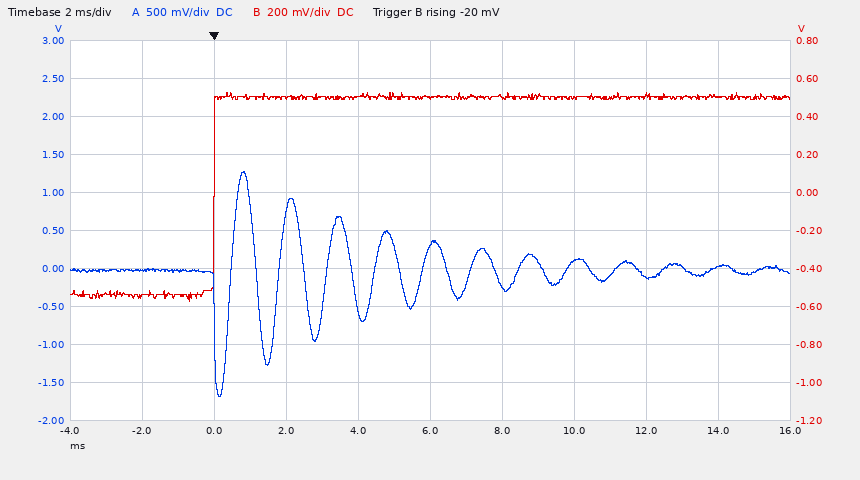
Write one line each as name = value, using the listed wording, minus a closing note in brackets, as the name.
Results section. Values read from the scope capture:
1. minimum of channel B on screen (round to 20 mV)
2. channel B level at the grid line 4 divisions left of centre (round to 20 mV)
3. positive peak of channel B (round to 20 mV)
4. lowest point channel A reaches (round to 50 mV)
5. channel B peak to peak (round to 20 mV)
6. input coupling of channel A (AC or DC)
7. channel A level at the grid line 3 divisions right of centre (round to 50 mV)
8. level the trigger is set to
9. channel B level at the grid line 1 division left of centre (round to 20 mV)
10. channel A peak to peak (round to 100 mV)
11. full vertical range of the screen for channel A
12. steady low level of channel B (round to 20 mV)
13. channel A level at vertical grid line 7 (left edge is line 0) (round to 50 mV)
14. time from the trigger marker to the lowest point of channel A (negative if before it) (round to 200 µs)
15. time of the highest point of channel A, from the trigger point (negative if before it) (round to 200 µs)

minimum of channel B on screen = -580 mV
channel B level at the grid line 4 divisions left of centre = -540 mV
positive peak of channel B = 520 mV
lowest point channel A reaches = -1.70 V
channel B peak to peak = 1.10 V
input coupling of channel A = DC
channel A level at the grid line 3 divisions right of centre = -100 mV
level the trigger is set to = -20 mV
channel B level at the grid line 1 division left of centre = 500 mV
channel A peak to peak = 3.00 V
full vertical range of the screen for channel A = 5 V
steady low level of channel B = -540 mV
channel A level at vertical grid line 7 (left edge is line 0) = 100 mV
time from the trigger marker to the lowest point of channel A (negative if before it) = +200 µs
time of the highest point of channel A, from the trigger point (negative if before it) = +800 µs
